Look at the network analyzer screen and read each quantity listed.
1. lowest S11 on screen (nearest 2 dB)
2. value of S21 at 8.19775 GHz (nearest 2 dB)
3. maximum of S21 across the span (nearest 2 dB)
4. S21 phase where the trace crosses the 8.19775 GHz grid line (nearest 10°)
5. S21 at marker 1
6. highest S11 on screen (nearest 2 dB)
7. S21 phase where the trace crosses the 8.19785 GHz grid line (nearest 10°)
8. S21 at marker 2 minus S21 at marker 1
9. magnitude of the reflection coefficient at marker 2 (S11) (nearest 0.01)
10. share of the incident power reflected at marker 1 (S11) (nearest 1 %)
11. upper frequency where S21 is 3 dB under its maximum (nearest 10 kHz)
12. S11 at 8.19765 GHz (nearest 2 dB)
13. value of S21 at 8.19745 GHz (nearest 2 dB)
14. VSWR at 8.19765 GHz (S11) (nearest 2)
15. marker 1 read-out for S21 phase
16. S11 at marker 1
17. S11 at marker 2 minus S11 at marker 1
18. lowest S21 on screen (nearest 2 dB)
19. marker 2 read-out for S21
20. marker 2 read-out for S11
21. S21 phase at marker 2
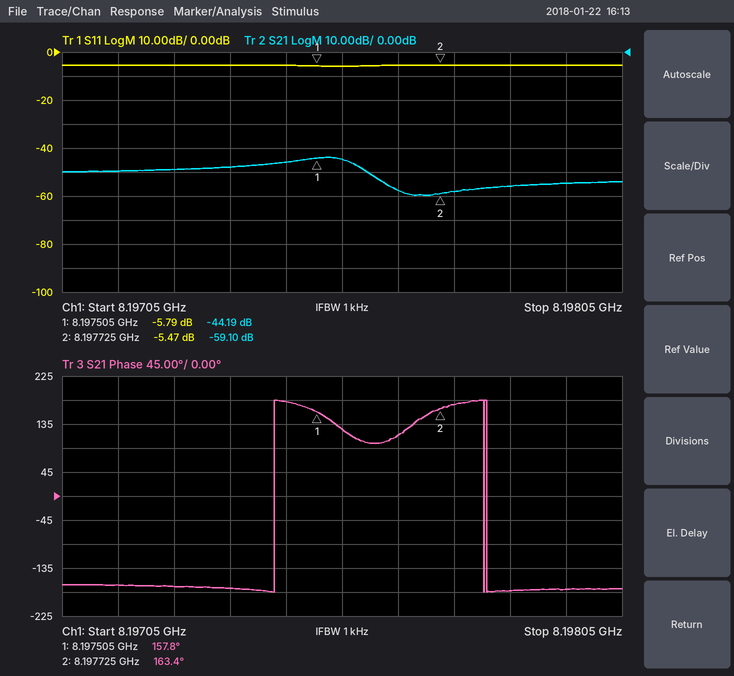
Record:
-6 dB
-58 dB
-44 dB
170°
-44.19 dB
-6 dB
-180°
-14.91 dB
0.53
26 %
8.19757 GHz
-6 dB
-46 dB
4
157.8°
-5.79 dB
0.32 dB
-60 dB
-59.10 dB
-5.47 dB
163.4°
